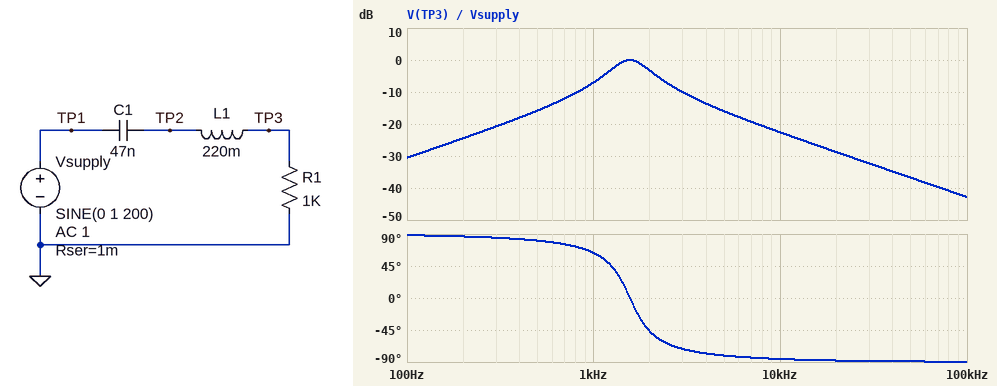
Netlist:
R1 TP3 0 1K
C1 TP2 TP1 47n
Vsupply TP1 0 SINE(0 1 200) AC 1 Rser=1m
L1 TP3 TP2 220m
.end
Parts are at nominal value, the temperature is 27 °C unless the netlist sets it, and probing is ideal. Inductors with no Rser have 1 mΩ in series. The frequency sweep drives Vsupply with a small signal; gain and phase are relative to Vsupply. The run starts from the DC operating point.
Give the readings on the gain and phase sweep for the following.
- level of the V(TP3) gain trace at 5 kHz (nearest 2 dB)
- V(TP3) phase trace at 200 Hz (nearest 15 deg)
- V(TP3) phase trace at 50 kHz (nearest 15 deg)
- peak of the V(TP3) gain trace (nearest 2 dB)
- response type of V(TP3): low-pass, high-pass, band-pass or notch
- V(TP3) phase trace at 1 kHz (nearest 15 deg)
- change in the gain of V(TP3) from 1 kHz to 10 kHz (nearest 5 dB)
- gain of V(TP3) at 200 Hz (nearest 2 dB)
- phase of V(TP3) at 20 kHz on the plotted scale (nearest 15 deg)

-16 dB
90 deg
-90 deg
0 dB
band-pass
60 deg
-15 dB
-24 dB
-90 deg
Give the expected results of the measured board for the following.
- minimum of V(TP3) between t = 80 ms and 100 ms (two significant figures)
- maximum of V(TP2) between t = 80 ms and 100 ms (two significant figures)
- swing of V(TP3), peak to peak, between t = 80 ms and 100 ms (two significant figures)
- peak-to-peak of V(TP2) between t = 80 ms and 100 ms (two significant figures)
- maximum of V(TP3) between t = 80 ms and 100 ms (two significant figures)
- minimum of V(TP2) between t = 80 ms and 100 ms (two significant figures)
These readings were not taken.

-60 mV
62 mV
120 mV
120 mV
60 mV
-62 mV
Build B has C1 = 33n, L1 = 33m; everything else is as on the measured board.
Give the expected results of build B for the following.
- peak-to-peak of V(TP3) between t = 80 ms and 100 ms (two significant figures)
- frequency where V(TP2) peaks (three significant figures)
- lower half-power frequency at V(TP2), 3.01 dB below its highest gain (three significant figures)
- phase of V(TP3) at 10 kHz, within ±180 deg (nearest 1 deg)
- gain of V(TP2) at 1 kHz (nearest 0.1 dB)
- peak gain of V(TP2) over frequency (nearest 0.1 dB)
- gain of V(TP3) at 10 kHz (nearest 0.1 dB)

83 mV
5.64 kHz
3.51 kHz
-58 deg
-13.3 dB
3.3 dB
-5.5 dB
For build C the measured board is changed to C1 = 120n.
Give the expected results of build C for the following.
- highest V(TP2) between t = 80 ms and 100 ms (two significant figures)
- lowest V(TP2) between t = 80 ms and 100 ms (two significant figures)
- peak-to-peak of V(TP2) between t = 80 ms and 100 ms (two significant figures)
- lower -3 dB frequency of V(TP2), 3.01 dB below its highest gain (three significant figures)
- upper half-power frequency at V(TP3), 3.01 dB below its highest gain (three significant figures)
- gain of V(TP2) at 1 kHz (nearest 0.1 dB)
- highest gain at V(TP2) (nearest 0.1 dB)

160 mV
-160 mV
320 mV
773 Hz
1.41 kHz
4.6 dB
4.8 dB
